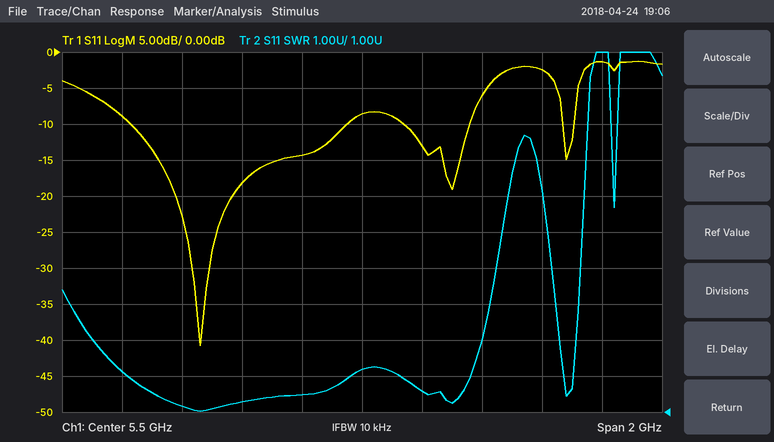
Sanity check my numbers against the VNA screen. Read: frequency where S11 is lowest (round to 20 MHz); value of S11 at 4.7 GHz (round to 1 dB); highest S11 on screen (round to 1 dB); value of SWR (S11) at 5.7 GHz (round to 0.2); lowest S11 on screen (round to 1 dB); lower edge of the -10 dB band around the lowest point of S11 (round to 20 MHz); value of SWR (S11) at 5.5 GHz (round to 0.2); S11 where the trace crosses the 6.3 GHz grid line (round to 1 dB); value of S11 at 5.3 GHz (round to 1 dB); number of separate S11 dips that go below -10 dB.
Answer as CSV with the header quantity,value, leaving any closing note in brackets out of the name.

quantity,value
frequency where S11 is lowest,4.96 GHz
value of S11 at 4.7 GHz,-9 dB
highest S11 on screen,-1 dB
value of SWR (S11) at 5.7 GHz,1.6
lowest S11 on screen,-41 dB
lower edge of the -10 dB band around the lowest point of S11,4.72 GHz
value of SWR (S11) at 5.5 GHz,2.2
S11 where the trace crosses the 6.3 GHz grid line,-1 dB
value of S11 at 5.3 GHz,-14 dB
number of separate S11 dips that go below -10 dB,3
